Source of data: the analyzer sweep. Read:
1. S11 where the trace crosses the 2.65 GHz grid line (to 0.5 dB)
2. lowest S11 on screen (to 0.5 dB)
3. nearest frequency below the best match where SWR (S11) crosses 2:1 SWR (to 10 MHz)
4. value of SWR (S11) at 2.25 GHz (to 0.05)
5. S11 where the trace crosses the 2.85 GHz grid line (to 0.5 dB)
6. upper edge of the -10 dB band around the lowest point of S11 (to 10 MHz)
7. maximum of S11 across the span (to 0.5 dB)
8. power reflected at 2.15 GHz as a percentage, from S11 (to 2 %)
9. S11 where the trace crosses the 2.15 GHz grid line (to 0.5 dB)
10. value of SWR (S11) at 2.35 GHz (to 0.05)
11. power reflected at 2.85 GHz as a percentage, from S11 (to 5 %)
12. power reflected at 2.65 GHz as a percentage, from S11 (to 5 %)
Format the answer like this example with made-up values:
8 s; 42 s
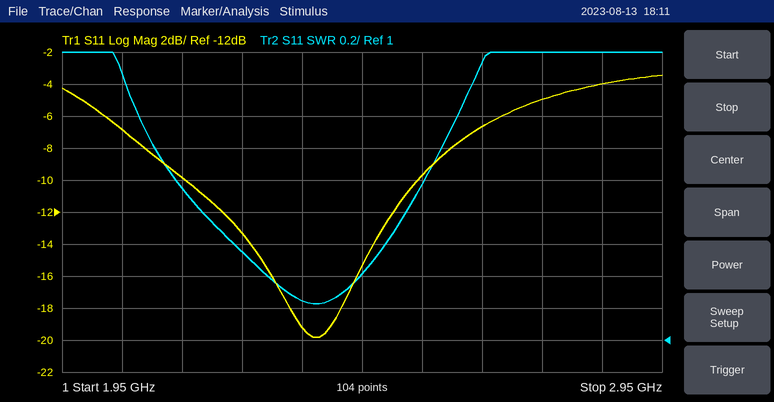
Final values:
-6.5 dB; -20.0 dB; 2.14 GHz; 1.55; -4.0 dB; 2.54 GHz; -3.5 dB; 10 %; -10.0 dB; 1.25; 40 %; 20 %
